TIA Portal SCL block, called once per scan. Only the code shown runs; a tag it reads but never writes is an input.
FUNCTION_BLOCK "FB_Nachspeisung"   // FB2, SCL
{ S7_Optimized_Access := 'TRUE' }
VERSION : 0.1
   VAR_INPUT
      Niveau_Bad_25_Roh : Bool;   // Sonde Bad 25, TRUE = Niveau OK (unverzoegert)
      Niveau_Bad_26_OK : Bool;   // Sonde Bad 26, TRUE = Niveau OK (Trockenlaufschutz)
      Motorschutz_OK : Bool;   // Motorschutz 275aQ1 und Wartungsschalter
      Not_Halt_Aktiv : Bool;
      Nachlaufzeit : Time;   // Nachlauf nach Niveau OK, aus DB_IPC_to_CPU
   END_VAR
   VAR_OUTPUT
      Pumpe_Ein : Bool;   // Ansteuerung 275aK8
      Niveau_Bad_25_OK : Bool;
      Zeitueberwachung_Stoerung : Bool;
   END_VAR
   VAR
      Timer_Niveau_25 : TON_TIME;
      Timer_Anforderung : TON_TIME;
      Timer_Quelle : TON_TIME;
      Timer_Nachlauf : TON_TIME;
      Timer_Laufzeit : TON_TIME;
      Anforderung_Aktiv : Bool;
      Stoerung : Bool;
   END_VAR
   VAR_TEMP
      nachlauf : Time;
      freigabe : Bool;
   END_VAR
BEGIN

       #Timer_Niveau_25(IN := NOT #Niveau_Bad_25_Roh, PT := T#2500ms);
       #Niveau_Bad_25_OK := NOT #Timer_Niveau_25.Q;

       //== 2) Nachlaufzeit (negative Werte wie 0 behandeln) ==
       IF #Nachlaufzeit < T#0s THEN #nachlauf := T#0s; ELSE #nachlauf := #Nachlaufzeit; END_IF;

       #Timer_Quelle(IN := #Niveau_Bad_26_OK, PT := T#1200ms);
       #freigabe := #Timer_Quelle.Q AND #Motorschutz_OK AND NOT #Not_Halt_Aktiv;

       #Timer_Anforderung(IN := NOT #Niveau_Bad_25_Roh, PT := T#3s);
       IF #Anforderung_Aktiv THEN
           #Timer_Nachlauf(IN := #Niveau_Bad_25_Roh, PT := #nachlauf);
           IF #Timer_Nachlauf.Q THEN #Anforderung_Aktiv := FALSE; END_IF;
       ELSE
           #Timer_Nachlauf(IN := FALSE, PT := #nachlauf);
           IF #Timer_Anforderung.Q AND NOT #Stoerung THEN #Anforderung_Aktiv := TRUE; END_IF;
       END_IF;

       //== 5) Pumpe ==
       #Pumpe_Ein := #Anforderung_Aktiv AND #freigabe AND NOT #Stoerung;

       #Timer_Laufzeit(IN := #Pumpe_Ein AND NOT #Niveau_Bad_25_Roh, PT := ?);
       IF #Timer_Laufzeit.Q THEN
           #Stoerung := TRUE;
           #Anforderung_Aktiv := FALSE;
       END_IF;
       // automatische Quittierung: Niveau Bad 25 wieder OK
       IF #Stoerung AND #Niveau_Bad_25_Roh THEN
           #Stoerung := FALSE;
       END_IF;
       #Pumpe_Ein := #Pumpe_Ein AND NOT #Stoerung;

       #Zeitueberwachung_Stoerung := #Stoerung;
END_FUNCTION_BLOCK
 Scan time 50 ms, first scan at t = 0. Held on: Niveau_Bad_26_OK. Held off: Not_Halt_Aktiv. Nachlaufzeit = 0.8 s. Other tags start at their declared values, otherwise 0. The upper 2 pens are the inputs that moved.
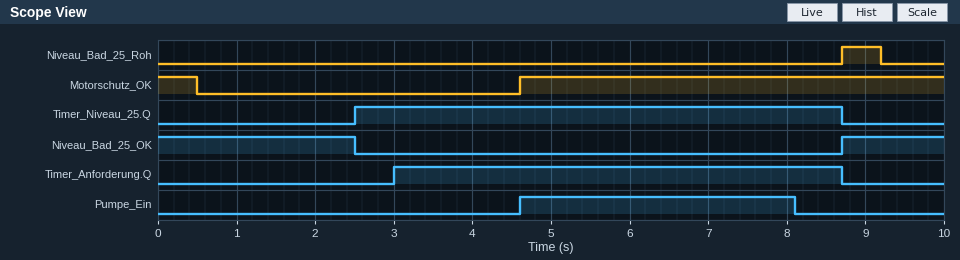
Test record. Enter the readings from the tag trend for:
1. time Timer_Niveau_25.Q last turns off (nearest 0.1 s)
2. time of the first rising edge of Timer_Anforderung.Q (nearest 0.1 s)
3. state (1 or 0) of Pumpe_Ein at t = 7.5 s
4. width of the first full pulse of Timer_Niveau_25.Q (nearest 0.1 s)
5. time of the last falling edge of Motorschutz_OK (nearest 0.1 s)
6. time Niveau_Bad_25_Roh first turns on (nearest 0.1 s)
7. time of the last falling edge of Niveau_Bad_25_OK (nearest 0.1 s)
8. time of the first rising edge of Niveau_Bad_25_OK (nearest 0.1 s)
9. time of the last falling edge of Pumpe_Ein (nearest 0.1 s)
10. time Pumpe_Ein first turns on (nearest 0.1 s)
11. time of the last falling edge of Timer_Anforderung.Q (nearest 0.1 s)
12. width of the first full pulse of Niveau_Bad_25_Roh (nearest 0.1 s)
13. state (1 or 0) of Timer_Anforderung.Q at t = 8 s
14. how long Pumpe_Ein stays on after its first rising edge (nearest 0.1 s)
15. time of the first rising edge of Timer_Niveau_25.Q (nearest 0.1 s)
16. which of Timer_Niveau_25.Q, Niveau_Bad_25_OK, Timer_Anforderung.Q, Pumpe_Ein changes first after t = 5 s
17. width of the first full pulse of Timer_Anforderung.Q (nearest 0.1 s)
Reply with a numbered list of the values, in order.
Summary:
1. 8.7 s
2. 3.0 s
3. 1
4. 6.2 s
5. 0.5 s
6. 8.7 s
7. 2.5 s
8. 8.7 s
9. 8.1 s
10. 4.6 s
11. 8.7 s
12. 0.5 s
13. 1
14. 3.5 s
15. 2.5 s
16. Pumpe_Ein
17. 5.7 s
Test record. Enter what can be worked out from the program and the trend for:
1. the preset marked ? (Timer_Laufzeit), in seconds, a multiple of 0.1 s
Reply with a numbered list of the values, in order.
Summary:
1. 3.5 s
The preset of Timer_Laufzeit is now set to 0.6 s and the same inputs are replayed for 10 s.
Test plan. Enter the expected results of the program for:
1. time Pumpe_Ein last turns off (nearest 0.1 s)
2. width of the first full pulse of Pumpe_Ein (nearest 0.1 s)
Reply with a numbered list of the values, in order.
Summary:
1. 5.2 s
2. 0.6 s
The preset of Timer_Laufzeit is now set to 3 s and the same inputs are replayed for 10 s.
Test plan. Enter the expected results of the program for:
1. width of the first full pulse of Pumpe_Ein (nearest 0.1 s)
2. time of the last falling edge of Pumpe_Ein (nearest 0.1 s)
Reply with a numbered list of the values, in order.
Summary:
1. 3.0 s
2. 7.6 s
